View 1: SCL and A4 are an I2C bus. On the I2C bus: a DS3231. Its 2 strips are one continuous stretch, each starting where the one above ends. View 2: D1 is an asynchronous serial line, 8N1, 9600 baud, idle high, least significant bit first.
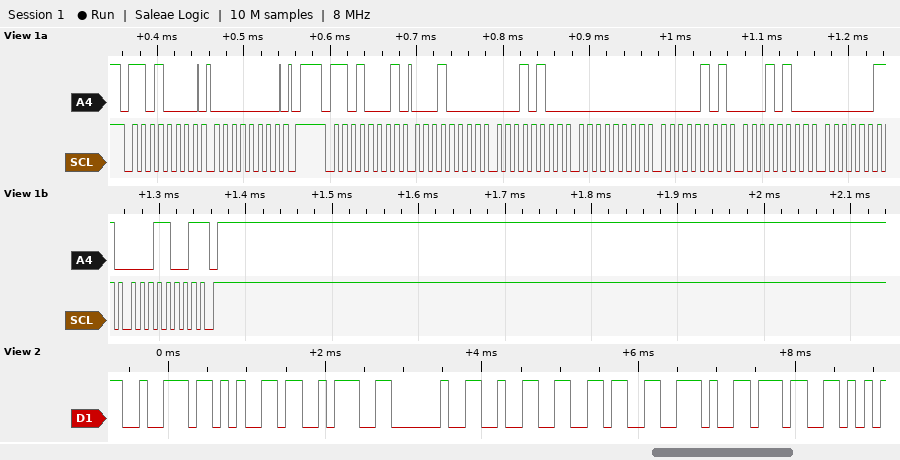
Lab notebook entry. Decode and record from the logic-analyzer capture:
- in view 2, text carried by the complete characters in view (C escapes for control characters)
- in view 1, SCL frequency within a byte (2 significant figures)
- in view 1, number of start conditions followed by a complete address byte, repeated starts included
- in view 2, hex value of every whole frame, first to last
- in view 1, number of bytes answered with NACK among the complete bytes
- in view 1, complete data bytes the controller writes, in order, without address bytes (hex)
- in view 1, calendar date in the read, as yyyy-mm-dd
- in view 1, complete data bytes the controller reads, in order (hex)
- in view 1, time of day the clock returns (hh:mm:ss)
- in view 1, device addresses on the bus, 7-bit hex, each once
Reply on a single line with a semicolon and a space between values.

"re: 26.7"; 100 kHz; 2; 72 65 3A 20 32 36 2E 37; 1; 00; 2019-03-14; 10 14 00 05 14 03 19; 00:14:10; 0x68
